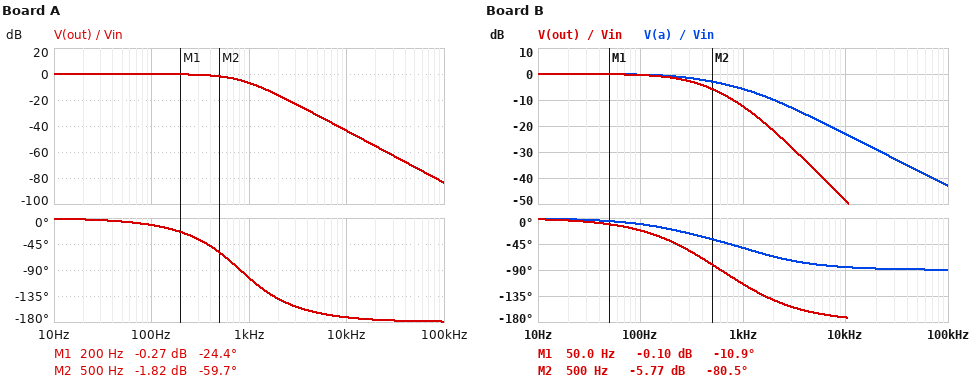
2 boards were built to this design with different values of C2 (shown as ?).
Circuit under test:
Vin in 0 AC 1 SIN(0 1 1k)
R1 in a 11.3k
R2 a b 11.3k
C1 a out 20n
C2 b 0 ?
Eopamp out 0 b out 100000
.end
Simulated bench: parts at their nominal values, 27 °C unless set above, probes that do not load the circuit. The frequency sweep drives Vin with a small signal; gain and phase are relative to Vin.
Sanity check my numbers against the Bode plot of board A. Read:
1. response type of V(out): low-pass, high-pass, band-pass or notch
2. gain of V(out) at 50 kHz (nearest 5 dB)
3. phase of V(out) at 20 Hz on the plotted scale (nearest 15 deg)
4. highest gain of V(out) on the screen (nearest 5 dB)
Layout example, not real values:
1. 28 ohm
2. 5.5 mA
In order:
1. low-pass
2. -70 dB
3. 0 deg
4. 0 dB
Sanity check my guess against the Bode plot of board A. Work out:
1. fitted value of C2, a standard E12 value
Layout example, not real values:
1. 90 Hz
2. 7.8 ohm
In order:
1. 15 nF
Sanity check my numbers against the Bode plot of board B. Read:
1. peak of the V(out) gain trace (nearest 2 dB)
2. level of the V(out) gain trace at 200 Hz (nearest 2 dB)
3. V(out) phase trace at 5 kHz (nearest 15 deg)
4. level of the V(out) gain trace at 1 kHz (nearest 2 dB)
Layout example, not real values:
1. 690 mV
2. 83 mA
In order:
1. 0 dB
2. -2 dB
3. -165 deg
4. -12 dB
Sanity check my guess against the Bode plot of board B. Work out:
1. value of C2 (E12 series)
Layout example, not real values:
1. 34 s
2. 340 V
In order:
1. 27 nF
